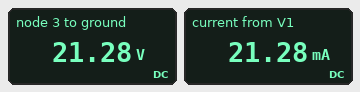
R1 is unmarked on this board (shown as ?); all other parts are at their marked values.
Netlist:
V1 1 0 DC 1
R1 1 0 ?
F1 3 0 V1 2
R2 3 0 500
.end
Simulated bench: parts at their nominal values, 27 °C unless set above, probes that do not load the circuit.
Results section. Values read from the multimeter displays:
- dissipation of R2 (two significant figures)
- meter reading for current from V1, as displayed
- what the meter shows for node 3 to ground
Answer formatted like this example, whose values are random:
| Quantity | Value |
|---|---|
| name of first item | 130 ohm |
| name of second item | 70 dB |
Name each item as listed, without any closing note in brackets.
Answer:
| Quantity | Value |
|---|---|
| dissipation of R2 | 910 mW |
| meter reading for current from V1, as displayed | 21.28 mA |
| what the meter shows for node 3 to ground | 21.28 V |
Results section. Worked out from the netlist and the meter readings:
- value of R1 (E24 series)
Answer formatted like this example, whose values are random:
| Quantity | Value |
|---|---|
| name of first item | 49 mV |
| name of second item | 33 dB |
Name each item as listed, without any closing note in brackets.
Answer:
| Quantity | Value |
|---|---|
| value of R1 | 47 Ω |
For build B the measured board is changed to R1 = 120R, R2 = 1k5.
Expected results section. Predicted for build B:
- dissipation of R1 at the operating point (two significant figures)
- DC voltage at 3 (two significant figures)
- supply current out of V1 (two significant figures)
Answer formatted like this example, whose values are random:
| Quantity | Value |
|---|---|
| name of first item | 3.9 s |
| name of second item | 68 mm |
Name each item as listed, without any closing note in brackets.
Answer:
| Quantity | Value |
|---|---|
| dissipation of R1 at the operating point | 8.3 mW |
| DC voltage at 3 | 25 V |
| supply current out of V1 | 8.3 mA |
